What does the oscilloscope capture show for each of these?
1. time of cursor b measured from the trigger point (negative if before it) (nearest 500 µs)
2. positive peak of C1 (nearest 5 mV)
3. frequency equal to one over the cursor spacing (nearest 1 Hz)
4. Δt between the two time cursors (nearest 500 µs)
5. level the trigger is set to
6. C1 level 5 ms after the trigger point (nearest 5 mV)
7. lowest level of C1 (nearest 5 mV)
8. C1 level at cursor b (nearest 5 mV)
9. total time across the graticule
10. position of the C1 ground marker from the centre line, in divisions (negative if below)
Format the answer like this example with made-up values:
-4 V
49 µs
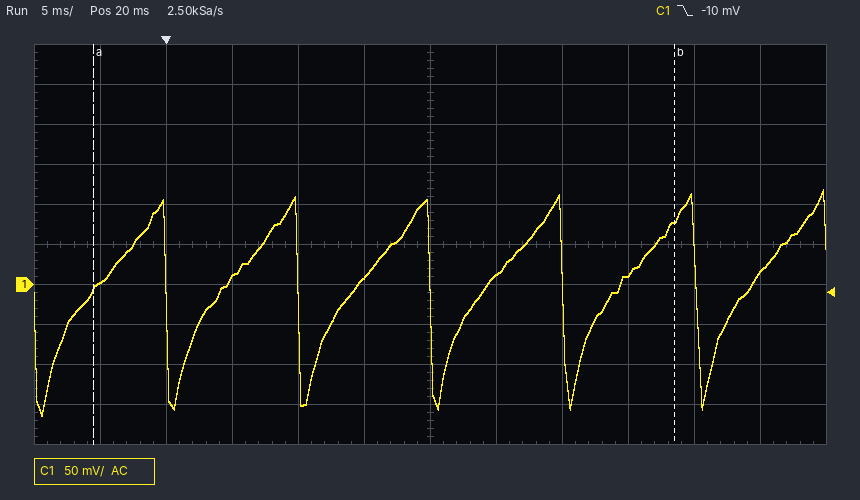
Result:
+38.5 ms
120 mV
23 Hz
44.0 ms
-10 mV
10 mV
-165 mV
80 mV
60 ms
-1.0 div
